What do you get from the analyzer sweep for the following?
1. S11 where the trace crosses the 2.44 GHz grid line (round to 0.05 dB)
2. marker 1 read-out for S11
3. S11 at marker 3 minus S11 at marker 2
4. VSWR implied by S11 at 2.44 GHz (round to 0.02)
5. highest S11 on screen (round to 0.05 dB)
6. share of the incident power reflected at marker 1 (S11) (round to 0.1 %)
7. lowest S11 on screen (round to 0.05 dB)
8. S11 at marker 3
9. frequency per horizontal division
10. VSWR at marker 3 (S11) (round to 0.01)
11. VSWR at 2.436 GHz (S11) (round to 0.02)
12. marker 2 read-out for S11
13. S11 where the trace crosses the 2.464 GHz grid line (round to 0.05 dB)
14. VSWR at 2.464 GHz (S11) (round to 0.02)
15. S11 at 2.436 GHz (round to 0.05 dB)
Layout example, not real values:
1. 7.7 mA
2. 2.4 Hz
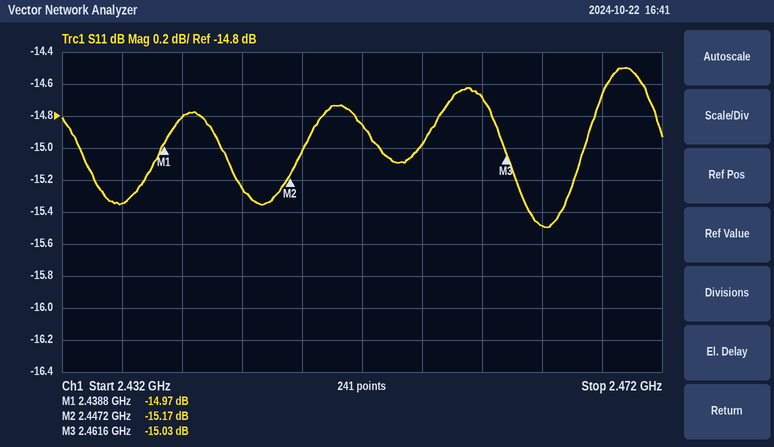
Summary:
1. -14.80 dB
2. -14.97 dB
3. 0.14 dB
4. 1.44
5. -14.50 dB
6. 3.2 %
7. -15.50 dB
8. -15.03 dB
9. 4 MHz
10. 1.43
11. 1.42
12. -15.17 dB
13. -15.50 dB
14. 1.40
15. -15.35 dB
